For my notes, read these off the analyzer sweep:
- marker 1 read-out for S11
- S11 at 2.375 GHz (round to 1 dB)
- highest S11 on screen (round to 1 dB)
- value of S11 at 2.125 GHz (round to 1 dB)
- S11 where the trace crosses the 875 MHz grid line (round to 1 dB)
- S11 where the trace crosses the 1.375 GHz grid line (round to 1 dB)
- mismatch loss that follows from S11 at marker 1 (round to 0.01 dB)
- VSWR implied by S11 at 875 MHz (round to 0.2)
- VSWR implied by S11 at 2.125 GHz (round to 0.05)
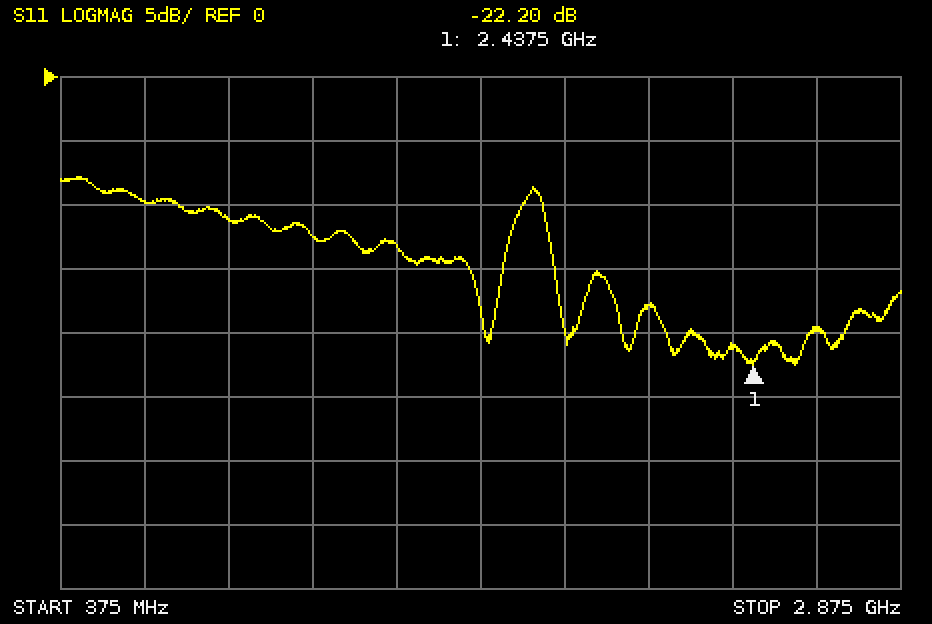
-22.20 dB
-21 dB
-8 dB
-18 dB
-11 dB
-13 dB
0.03 dB
1.8
1.30
